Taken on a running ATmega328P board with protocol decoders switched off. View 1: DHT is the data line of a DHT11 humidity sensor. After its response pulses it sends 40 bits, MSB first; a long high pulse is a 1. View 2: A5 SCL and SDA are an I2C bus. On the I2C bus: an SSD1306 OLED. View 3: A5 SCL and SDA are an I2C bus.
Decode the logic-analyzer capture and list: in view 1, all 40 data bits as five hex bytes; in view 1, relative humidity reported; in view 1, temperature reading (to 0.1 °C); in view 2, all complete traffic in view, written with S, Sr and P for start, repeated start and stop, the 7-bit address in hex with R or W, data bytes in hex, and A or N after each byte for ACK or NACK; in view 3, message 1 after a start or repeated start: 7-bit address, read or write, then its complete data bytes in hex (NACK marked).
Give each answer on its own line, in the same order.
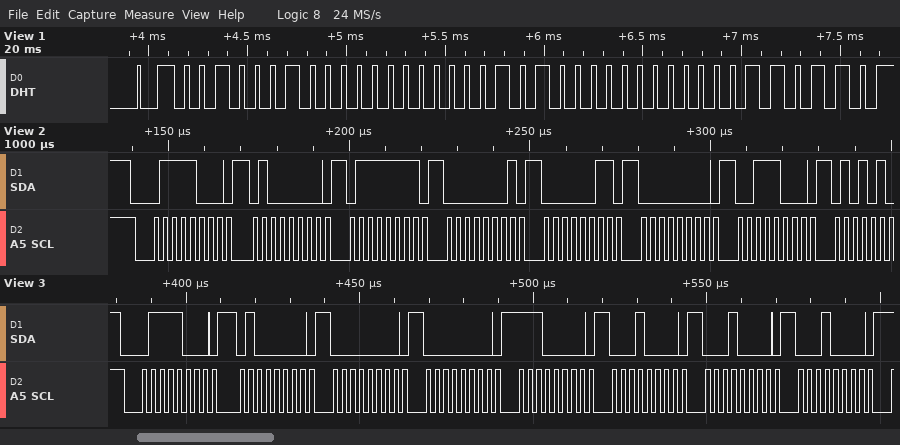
22 00 14 00 36
34 %
20.0 °C
S 3CW A 40 A 7F A 01 A 03 A 00 A 38 A
0x3C write: 40 00 00 E0 10 10 10
